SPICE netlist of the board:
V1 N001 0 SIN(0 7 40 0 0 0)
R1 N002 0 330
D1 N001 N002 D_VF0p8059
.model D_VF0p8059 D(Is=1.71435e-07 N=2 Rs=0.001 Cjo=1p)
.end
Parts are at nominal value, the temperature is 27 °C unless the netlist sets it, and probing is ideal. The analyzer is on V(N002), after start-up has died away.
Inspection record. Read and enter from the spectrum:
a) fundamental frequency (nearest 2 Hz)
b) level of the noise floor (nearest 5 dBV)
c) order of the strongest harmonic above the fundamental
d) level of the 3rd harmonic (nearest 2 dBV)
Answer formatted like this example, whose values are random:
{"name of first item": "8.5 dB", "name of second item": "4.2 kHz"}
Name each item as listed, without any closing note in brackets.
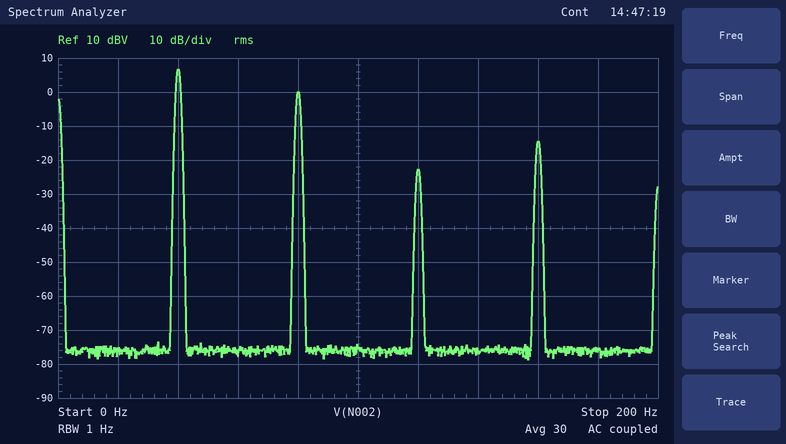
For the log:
{"fundamental frequency": "40 Hz", "level of the noise floor": "-75 dBV", "order of the strongest harmonic above the fundamental": "2", "level of the 3rd harmonic": "-22 dBV"}
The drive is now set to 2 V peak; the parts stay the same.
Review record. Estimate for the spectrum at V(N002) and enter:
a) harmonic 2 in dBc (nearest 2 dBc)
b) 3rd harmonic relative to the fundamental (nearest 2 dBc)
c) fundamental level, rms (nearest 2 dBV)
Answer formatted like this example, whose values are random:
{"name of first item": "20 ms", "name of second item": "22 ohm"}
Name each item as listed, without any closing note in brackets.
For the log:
{"harmonic 2 in dBc": "-6 dBc", "3rd harmonic relative to the fundamental": "-18 dBc", "fundamental level, rms": "-6 dBV"}
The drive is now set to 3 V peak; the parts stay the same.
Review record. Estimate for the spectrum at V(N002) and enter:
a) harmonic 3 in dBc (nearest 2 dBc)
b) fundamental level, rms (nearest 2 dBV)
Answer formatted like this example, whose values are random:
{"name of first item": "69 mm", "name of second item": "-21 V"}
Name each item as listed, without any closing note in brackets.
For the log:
{"harmonic 3 in dBc": "-22 dBc", "fundamental level, rms": "-2 dBV"}
